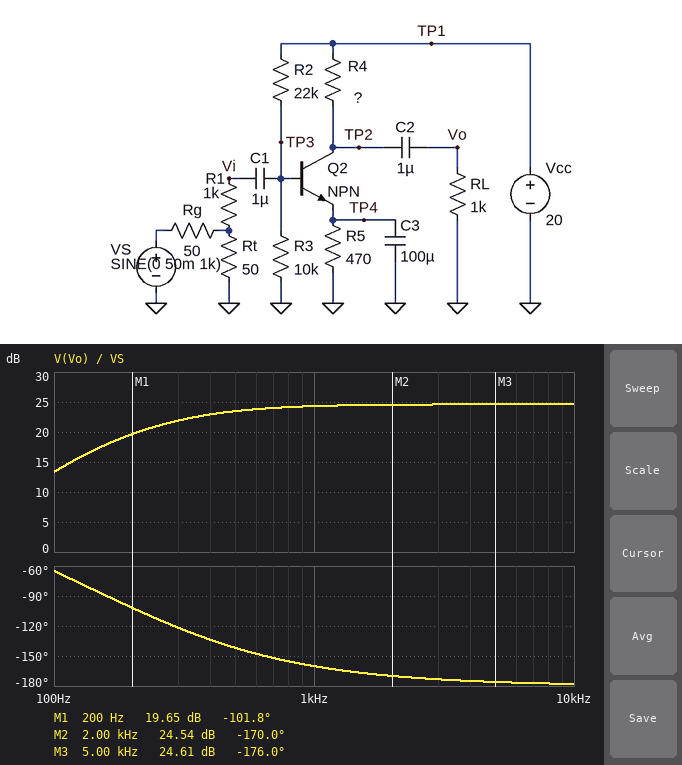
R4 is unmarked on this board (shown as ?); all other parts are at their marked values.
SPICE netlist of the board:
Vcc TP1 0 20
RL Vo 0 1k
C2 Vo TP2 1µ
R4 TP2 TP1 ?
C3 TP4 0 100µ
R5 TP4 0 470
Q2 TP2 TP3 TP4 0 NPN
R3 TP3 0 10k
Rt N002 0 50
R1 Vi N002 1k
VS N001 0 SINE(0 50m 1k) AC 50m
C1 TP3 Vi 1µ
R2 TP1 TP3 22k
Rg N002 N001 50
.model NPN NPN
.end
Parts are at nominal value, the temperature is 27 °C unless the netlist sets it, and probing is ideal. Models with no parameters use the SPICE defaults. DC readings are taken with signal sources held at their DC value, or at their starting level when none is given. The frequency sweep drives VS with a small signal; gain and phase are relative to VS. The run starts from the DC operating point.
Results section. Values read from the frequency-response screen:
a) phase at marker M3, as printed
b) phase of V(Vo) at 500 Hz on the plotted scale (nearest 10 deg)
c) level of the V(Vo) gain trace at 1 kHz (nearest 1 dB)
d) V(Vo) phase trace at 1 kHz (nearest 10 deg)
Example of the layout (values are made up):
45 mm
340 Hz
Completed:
-176.0 deg
-140 deg
24 dB
-160 deg
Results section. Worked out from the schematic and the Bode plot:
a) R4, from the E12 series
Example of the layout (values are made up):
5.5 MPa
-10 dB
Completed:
820 Ω
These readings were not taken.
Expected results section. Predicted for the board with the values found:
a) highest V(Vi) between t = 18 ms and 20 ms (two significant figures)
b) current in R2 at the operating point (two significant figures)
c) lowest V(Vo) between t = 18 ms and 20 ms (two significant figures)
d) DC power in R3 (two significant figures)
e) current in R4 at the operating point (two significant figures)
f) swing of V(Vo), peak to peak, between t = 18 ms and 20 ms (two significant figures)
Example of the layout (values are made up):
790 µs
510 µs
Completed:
7.7 mV
660 µA
-830 mV
3.1 mW
10 mA
1.6 V
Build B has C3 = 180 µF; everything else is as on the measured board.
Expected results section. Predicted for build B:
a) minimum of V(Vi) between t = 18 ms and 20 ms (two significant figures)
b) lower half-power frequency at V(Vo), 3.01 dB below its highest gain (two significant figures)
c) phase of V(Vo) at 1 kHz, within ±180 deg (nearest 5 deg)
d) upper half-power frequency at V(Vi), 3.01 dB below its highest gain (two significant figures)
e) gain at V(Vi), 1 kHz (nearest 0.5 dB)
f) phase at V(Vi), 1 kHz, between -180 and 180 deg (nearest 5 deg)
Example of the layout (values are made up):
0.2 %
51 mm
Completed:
-6.7 mV
230 Hz
-165 deg
190 Hz
-17.5 dB
-35 deg
